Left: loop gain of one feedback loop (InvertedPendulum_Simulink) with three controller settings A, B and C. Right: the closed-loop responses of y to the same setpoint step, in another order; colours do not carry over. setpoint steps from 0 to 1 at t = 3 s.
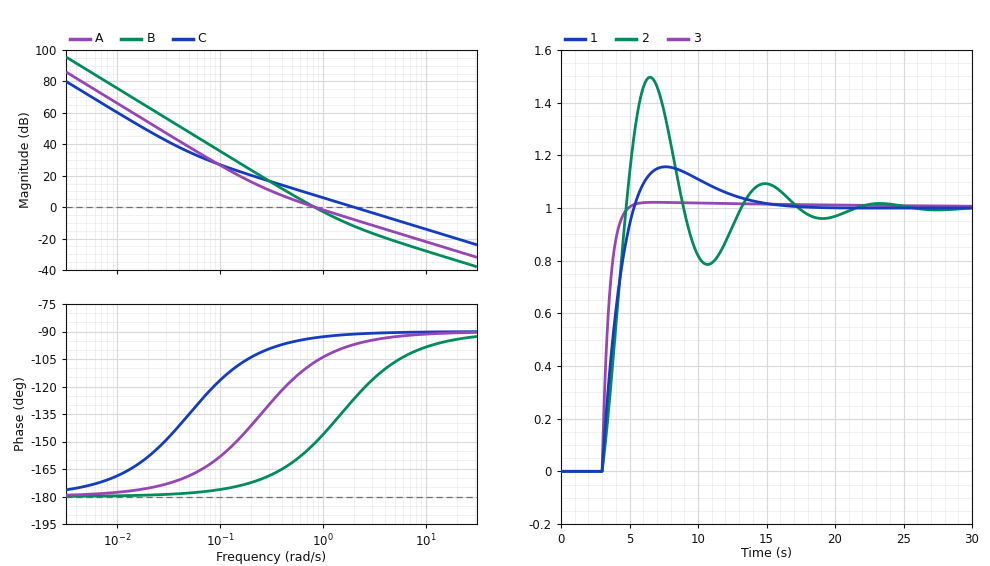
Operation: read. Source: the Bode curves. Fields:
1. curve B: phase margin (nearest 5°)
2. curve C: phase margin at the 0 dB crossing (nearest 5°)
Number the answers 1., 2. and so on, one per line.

1. 30°
2. 90°
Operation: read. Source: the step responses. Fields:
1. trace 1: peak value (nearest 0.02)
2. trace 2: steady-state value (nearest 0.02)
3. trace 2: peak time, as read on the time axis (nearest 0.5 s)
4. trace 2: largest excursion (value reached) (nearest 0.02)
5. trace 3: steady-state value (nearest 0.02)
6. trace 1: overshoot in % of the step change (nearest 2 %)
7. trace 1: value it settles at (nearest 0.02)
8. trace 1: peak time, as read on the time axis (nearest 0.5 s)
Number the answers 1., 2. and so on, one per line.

1. 1.16
2. 1.00
3. 6.5 s
4. 1.50
5. 1.00
6. 16 %
7. 1.00
8. 7.5 s
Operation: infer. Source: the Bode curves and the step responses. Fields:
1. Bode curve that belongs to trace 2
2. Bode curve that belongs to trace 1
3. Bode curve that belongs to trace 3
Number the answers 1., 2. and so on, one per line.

1. B
2. A
3. C
